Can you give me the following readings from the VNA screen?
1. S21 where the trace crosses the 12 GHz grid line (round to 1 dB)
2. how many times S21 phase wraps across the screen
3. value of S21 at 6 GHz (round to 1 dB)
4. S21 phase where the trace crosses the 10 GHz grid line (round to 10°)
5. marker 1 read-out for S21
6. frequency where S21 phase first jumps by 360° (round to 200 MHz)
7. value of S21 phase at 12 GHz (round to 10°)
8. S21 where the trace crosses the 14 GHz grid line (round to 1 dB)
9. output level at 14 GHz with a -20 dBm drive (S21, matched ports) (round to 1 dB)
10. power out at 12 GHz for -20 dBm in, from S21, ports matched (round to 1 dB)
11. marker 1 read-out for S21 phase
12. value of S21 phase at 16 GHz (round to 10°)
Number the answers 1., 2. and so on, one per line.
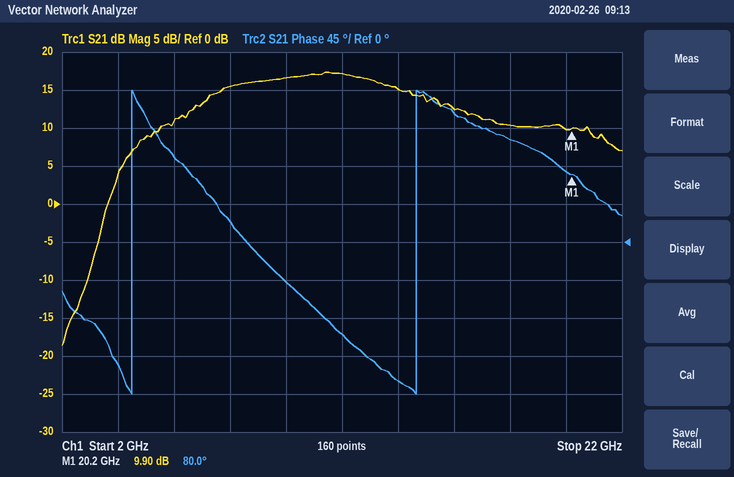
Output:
1. 17 dB
2. 2
3. 11 dB
4. -50°
5. 9.90 dB
6. 4.4 GHz
7. -110°
8. 15 dB
9. -5 dBm
10. -3 dBm
11. 80.0°
12. 150°
